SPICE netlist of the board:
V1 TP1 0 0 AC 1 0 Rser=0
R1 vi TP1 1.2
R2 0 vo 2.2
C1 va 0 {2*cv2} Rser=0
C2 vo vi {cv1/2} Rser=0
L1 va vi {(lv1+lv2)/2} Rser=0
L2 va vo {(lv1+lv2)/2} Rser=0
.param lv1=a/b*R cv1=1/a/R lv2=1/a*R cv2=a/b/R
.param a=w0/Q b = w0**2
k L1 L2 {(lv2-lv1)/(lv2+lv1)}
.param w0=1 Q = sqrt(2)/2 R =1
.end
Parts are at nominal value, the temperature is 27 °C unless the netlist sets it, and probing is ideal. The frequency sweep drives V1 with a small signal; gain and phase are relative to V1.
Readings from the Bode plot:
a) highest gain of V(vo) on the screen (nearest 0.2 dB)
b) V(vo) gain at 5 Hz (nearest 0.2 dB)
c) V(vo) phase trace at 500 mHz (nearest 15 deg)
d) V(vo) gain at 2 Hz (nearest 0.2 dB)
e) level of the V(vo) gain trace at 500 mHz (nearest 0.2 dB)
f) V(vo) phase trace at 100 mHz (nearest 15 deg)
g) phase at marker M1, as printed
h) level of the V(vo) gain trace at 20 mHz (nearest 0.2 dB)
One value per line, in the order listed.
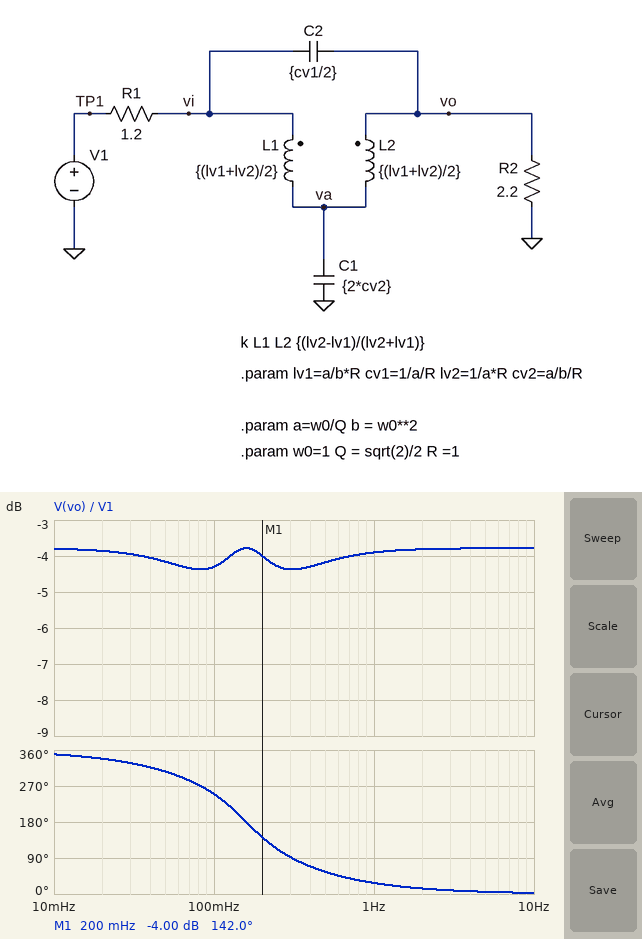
-3.8 dB
-3.8 dB
60 deg
-3.8 dB
-4.2 dB
255 deg
142.0 deg
-3.8 dB
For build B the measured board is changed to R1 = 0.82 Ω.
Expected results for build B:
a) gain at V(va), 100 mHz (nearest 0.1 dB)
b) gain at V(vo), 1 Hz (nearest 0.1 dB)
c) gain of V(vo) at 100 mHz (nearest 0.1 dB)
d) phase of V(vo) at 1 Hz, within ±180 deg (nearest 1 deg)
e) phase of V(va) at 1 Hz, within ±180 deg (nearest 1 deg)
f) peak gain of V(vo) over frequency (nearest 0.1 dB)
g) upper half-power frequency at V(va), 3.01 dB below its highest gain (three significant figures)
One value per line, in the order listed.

-6.2 dB
-2.6 dB
-2.2 dB
24 deg
-162 deg
-2.1 dB
95.6 mHz
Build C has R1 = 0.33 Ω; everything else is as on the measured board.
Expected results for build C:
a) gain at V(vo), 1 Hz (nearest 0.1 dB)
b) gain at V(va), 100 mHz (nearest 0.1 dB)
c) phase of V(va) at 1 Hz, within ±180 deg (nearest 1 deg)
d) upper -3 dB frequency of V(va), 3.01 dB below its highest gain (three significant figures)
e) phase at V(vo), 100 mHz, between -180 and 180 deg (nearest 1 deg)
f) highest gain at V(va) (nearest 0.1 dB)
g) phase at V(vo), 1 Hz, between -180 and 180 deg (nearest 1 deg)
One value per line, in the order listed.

-0.7 dB
-2.5 dB
-168 deg
102 mHz
-120 deg
0.1 dB
18 deg
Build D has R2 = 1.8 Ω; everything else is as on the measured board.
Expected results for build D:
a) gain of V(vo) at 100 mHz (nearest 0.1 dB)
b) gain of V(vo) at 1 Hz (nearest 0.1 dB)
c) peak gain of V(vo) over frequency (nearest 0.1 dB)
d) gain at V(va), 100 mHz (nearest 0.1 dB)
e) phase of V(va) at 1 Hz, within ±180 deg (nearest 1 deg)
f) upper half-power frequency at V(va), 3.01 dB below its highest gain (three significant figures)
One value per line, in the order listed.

-4.8 dB
-4.5 dB
-4.4 dB
-8.2 dB
-160 deg
88.8 mHz
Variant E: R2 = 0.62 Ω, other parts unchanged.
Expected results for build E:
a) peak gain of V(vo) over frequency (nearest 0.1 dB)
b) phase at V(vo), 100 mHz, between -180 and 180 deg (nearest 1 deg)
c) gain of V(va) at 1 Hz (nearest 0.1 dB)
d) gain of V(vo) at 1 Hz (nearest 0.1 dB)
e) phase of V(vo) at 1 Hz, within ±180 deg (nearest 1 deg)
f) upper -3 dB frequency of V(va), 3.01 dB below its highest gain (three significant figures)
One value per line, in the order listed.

-9.0 dB
-112 deg
-40.9 dB
-9.3 dB
25 deg
180 mHz
